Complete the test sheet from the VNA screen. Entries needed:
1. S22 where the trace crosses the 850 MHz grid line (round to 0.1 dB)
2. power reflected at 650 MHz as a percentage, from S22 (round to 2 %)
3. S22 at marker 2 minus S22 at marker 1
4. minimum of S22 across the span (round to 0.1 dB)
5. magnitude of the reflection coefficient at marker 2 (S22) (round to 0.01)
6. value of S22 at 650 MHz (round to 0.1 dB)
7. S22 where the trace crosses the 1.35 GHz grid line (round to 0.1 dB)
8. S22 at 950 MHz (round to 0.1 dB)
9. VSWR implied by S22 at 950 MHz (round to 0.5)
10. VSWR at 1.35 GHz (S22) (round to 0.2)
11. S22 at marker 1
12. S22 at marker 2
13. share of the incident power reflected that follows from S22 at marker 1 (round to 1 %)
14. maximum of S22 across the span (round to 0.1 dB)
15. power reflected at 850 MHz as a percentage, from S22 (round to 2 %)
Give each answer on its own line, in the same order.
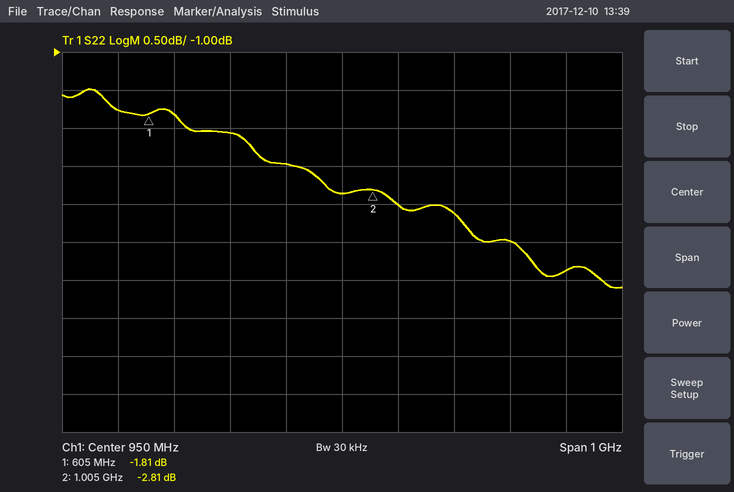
-2.5 dB
66 %
-1.00 dB
-4.1 dB
0.72
-1.8 dB
-3.9 dB
-2.9 dB
6.0
4.6
-1.81 dB
-2.81 dB
66 %
-1.5 dB
56 %
